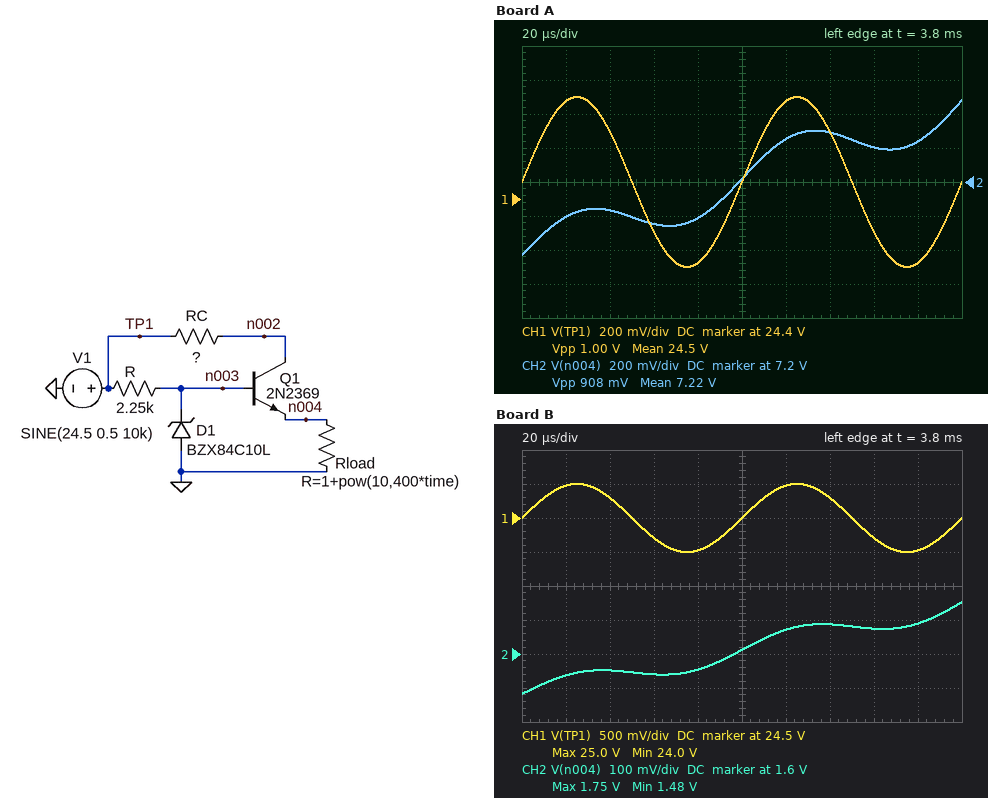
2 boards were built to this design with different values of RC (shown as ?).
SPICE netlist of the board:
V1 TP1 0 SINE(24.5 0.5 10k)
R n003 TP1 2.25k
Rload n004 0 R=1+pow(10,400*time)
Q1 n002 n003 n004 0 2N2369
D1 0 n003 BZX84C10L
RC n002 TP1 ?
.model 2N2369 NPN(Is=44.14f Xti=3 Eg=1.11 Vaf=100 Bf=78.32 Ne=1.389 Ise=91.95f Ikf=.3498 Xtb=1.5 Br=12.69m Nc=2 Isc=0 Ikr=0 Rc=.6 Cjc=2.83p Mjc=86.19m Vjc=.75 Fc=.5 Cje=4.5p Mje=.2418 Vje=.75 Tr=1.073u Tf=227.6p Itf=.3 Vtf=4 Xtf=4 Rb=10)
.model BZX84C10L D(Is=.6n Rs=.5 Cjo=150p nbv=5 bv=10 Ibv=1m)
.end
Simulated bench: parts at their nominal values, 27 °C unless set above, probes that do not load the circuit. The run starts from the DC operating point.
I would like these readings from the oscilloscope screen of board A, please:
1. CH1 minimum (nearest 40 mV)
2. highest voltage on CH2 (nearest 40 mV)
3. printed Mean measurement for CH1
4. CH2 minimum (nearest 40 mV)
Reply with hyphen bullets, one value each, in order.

- 24.00 V
- 7.68 V
- 24.5 V
- 6.76 V
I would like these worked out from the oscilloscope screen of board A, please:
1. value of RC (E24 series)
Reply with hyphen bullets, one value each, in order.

- 91 Ω
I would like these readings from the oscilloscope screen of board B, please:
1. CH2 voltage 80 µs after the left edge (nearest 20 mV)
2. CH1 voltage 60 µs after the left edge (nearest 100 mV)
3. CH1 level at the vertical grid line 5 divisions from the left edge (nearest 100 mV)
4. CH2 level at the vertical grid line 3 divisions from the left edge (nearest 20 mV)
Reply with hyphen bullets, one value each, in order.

- 1.56 V
- 24.2 V
- 24.5 V
- 1.54 V
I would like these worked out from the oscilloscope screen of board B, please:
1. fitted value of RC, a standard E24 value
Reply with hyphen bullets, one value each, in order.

- 680 Ω
